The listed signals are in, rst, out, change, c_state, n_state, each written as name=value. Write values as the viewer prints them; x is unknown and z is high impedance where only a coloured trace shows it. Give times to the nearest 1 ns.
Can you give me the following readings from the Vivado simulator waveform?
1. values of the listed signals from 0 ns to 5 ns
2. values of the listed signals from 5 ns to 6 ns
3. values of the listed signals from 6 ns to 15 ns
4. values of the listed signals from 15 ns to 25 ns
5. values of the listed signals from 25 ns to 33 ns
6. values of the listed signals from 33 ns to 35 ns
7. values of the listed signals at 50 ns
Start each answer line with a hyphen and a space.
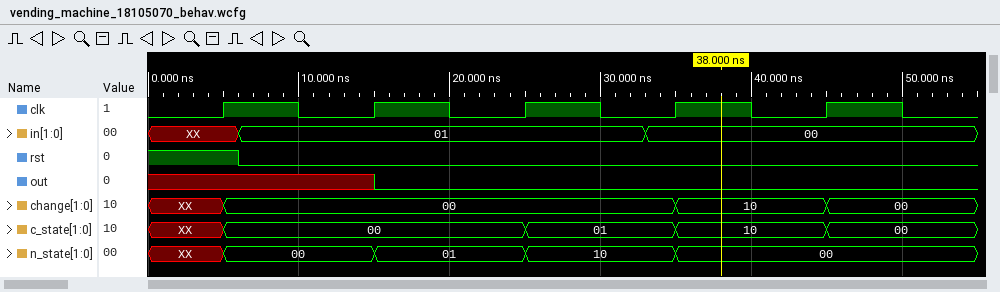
- in=XX, rst=1, out=x, change=XX, c_state=XX, n_state=XX
- in=XX, rst=1, out=x, change=00, c_state=00, n_state=00
- in=01, rst=0, out=x, change=00, c_state=00, n_state=00
- in=01, rst=0, out=0, change=00, c_state=00, n_state=01
- in=01, rst=0, out=0, change=00, c_state=01, n_state=10
- in=00, rst=0, out=0, change=00, c_state=01, n_state=10
- in=00, rst=0, out=0, change=00, c_state=00, n_state=00
